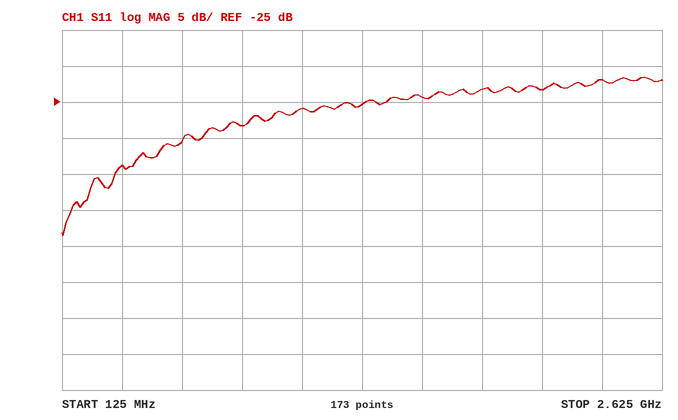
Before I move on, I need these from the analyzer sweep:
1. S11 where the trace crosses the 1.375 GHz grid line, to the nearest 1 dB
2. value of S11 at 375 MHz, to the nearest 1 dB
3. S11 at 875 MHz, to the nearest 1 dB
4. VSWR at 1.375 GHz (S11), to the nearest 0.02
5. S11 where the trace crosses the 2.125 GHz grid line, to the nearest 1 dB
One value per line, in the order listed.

-25 dB
-34 dB
-28 dB
1.12
-23 dB
